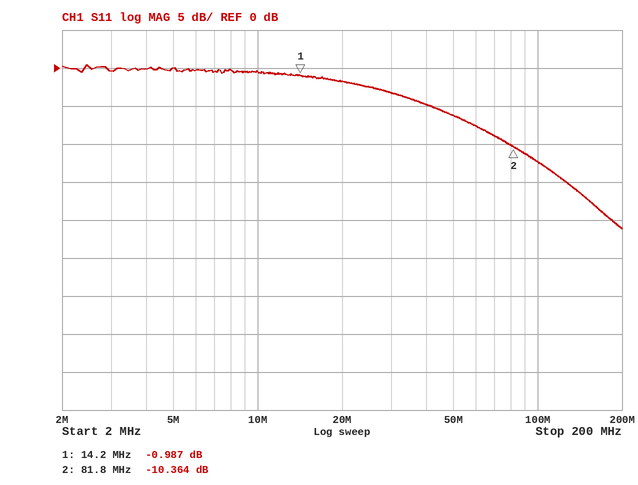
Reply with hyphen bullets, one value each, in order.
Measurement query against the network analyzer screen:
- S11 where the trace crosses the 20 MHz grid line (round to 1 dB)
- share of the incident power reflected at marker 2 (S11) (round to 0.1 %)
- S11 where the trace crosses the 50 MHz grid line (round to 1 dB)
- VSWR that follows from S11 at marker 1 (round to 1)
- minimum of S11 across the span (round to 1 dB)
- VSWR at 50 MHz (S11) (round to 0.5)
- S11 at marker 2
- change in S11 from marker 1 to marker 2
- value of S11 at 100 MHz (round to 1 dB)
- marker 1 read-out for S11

- -2 dB
- 9.2 %
- -6 dB
- 18
- -21 dB
- 3.0
- -10.364 dB
- -9.377 dB
- -12 dB
- -0.987 dB
